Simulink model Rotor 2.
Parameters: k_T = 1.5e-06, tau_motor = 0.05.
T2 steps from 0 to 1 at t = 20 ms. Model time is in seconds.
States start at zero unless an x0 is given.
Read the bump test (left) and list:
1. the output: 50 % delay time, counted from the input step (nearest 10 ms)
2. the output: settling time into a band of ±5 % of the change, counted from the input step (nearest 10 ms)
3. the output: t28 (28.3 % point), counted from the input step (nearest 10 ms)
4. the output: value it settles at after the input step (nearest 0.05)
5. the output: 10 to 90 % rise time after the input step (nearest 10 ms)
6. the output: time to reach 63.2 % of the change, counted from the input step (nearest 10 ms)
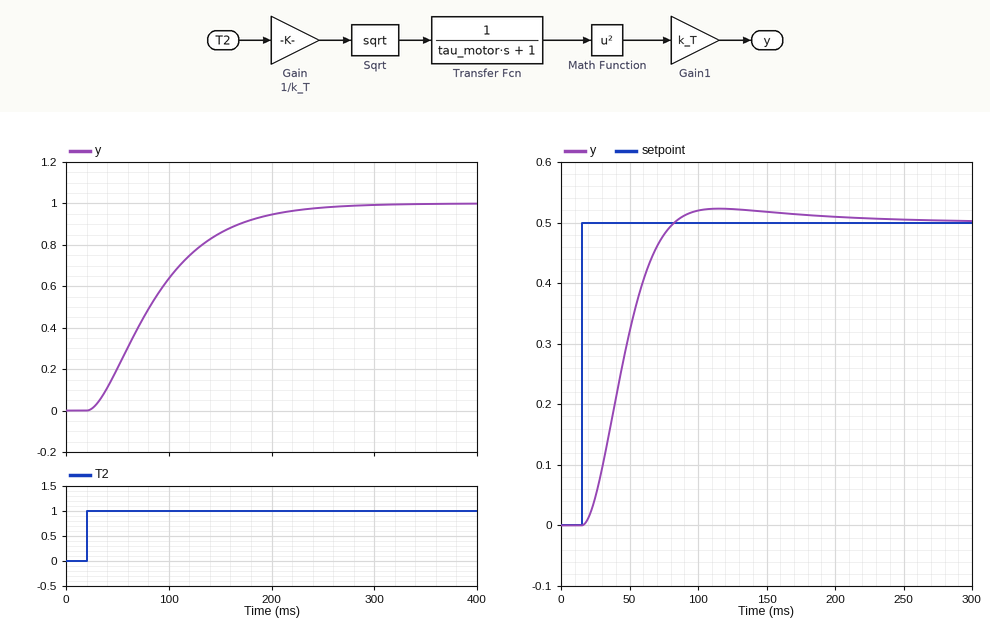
60 ms
180 ms
40 ms
1.00
130 ms
80 ms
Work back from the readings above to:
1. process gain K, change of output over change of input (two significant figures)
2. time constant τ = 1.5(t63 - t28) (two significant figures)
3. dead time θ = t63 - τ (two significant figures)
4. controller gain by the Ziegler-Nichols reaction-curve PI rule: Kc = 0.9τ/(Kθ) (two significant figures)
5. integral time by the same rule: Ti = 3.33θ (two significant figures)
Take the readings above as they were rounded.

1.0
60 ms
20 ms
2.7
67 ms
